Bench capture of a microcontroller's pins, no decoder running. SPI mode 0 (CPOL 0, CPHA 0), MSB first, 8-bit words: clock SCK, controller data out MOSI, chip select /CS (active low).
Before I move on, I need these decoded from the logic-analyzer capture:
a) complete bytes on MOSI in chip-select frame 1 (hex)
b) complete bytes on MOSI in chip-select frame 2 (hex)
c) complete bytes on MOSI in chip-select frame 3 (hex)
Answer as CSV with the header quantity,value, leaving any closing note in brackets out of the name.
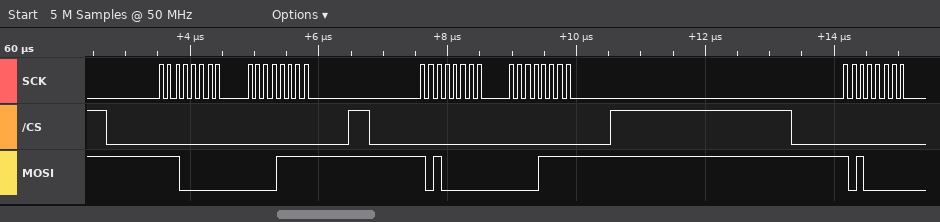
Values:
quantity,value
complete bytes on MOSI in chip-select frame 1,E0 0F
complete bytes on MOSI in chip-select frame 2,A0 0F
complete bytes on MOSI in chip-select frame 3,A0
